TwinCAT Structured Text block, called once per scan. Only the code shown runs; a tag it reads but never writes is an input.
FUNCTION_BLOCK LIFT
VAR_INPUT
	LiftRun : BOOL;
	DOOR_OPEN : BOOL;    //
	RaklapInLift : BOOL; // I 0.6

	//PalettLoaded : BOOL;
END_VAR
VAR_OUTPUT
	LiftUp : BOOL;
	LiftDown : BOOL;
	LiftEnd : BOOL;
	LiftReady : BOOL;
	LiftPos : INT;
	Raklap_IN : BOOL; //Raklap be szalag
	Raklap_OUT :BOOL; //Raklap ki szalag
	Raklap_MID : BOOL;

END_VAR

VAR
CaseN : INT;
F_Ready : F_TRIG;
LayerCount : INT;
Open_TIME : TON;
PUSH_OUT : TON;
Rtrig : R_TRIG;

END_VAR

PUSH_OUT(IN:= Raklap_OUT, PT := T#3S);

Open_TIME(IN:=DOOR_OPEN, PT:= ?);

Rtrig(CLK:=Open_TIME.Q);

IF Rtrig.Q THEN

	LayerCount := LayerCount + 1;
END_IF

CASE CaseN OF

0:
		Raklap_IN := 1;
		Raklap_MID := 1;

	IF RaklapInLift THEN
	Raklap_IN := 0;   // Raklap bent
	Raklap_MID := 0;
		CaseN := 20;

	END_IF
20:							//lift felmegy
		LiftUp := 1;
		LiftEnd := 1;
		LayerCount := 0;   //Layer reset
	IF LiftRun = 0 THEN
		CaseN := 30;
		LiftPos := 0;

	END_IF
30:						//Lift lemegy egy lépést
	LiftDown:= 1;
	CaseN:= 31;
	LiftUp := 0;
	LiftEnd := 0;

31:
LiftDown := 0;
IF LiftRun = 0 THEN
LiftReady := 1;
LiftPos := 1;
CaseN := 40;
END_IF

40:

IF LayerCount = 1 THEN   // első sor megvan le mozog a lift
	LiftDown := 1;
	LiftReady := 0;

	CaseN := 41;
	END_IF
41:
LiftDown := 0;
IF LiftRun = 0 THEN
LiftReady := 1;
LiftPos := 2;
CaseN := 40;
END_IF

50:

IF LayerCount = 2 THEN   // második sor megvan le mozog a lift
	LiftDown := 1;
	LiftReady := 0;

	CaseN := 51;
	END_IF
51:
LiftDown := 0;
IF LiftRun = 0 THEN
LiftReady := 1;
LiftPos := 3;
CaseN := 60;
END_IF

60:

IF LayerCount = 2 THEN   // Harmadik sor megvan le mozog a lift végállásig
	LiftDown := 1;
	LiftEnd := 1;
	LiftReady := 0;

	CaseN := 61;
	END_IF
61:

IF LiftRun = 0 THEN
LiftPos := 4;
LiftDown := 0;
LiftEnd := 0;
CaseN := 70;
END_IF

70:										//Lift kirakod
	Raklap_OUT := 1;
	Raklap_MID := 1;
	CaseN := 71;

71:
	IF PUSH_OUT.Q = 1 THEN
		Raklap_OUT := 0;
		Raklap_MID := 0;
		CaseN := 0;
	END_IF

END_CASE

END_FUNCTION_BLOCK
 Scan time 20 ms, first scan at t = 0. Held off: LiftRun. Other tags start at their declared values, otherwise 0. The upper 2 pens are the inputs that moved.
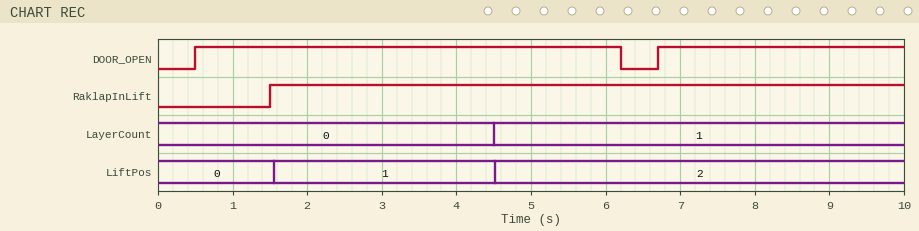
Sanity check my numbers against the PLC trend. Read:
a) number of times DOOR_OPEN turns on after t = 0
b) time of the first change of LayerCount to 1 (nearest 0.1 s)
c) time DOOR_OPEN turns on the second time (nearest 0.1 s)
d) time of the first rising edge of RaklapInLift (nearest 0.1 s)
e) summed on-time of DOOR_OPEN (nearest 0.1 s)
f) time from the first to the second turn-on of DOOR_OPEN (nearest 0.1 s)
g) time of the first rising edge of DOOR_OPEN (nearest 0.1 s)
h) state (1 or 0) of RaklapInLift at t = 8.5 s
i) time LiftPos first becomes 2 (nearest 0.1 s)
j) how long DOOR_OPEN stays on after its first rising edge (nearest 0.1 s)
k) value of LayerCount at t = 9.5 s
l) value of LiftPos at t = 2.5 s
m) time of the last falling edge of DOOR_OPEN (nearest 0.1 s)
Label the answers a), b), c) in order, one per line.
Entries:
a) 2
b) 4.5 s
c) 6.7 s
d) 1.5 s
e) 9.0 s
f) 6.2 s
g) 0.5 s
h) 1
i) 4.5 s
j) 5.7 s
k) 1
l) 1
m) 6.2 s
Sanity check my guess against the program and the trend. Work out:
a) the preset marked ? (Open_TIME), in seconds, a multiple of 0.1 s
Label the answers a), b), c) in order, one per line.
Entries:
a) 4.0 s
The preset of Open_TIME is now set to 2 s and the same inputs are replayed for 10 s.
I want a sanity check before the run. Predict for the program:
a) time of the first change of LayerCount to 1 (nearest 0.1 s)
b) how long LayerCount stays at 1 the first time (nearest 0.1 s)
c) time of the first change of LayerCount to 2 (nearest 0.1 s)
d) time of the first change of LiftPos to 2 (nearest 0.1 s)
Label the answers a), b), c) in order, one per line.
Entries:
a) 2.5 s
b) 6.2 s
c) 8.7 s
d) 2.5 s
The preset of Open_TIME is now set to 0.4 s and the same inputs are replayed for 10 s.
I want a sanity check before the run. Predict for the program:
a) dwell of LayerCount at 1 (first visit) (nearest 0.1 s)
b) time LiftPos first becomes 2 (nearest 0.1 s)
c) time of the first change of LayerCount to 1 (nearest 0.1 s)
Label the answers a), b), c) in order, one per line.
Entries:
a) 0.6 s
b) 7.1 s
c) 0.9 s
